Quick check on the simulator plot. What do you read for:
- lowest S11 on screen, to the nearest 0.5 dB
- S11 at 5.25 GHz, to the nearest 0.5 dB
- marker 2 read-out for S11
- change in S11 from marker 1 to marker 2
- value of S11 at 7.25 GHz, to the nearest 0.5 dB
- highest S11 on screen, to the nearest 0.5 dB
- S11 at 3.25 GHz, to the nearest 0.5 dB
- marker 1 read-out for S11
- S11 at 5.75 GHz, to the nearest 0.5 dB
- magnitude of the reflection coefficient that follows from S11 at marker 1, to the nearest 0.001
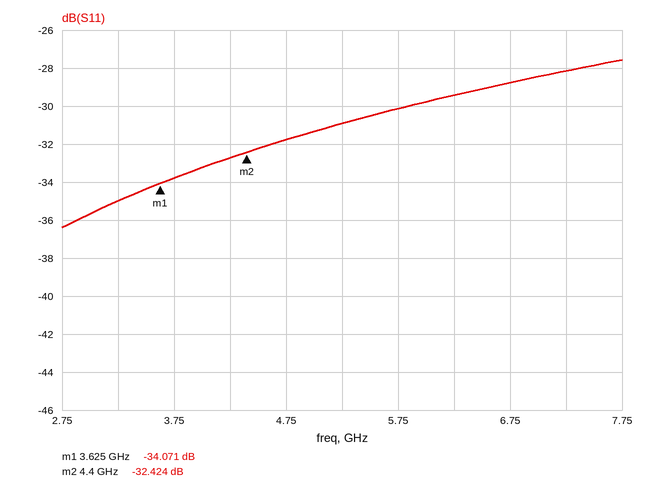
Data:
-36.5 dB
-31.0 dB
-32.424 dB
1.647 dB
-28.0 dB
-27.5 dB
-35.0 dB
-34.071 dB
-30.0 dB
0.020
